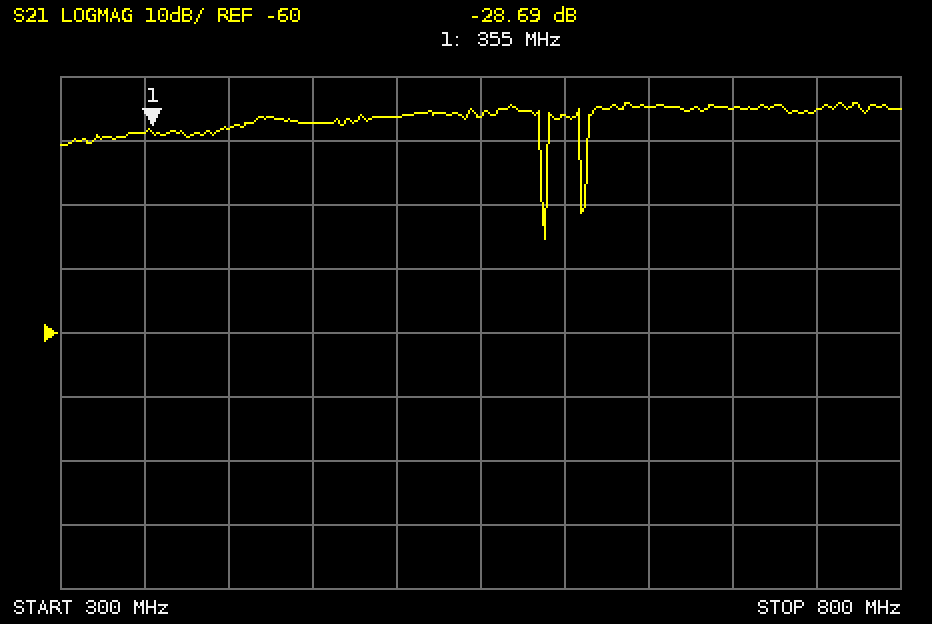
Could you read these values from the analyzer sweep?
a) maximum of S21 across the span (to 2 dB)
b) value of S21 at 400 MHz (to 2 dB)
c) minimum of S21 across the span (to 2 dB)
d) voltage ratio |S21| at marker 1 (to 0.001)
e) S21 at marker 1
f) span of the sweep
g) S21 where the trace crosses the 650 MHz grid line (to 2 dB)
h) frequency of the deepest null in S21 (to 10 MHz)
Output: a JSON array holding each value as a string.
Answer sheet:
["-24 dB", "-28 dB", "-46 dB", "0.037", "-28.69 dB", "500 MHz", "-24 dB", "590 MHz"]
